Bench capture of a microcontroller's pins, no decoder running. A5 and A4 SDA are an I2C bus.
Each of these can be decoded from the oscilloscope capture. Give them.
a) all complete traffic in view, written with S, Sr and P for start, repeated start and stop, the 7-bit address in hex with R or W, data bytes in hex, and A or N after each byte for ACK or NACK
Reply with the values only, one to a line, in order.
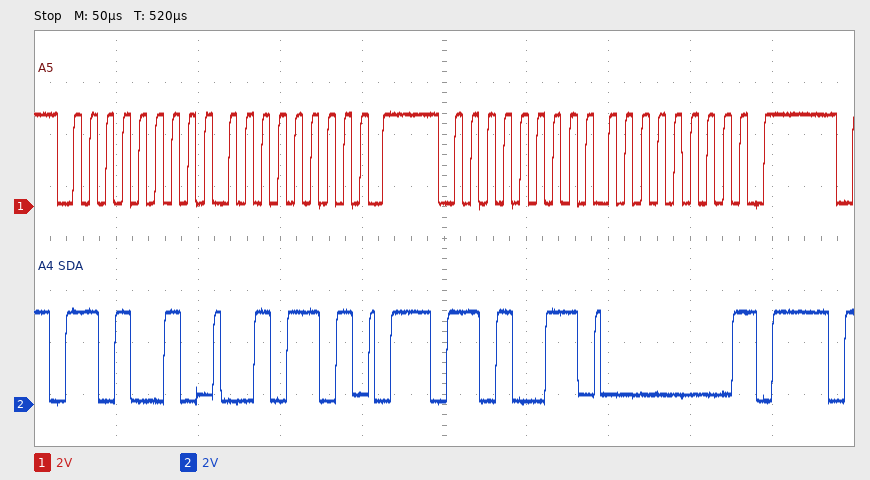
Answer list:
S 69W A 2D A P S 69R A 00 N P
